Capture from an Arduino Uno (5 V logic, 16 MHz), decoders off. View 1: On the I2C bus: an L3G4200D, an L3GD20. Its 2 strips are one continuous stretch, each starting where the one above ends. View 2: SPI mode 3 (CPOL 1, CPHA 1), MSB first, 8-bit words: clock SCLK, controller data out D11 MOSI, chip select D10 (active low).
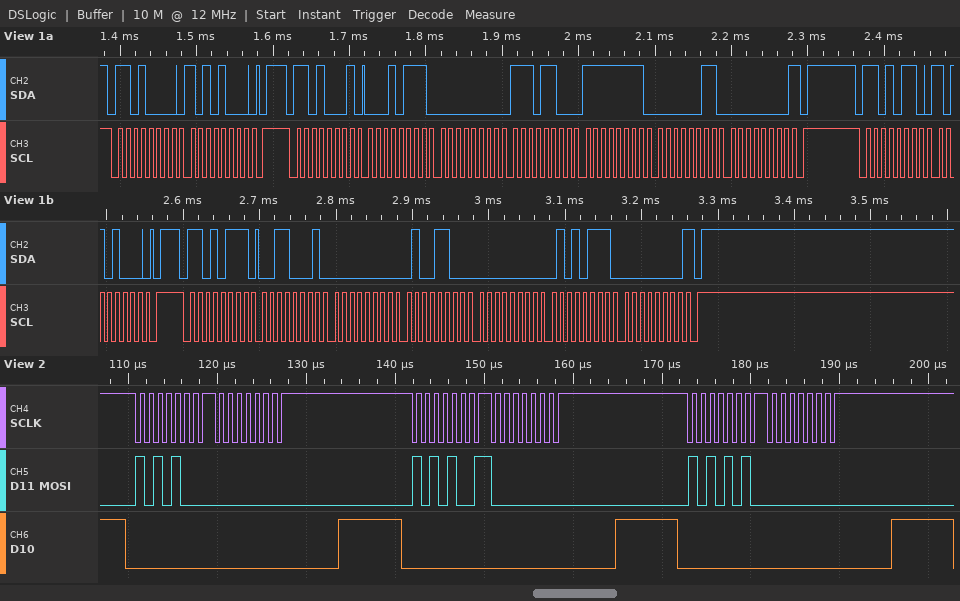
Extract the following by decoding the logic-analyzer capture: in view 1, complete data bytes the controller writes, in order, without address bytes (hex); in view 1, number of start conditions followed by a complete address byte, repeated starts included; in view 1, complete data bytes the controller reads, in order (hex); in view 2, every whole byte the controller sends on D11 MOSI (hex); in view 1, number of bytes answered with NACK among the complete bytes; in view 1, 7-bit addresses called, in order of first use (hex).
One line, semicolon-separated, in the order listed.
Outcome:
A8 A8; 4; 17 00 EC FF 03 00 31 00 4C 00 57 00; A8 00 A9 00 AA 00; 2; 0x68 0x6B
